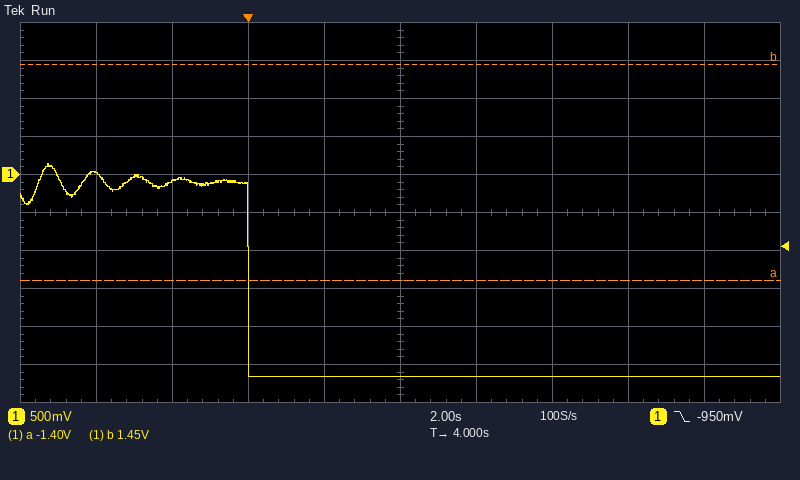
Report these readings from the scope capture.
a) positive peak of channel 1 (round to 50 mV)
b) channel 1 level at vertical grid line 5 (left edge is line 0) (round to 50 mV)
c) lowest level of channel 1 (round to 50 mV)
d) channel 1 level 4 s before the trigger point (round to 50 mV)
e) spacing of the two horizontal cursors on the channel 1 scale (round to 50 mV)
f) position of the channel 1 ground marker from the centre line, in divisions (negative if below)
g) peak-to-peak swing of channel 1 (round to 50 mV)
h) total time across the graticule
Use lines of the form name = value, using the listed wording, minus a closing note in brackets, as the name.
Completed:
positive peak of channel 1 = 150 mV
channel 1 level at vertical grid line 5 (left edge is line 0) = -2.65 V
lowest level of channel 1 = -2.65 V
channel 1 level 4 s before the trigger point = 0 mV
spacing of the two horizontal cursors on the channel 1 scale = 2.85 V
position of the channel 1 ground marker from the centre line, in divisions = +1.0 div
peak-to-peak swing of channel 1 = 2.80 V
total time across the graticule = 20 s
